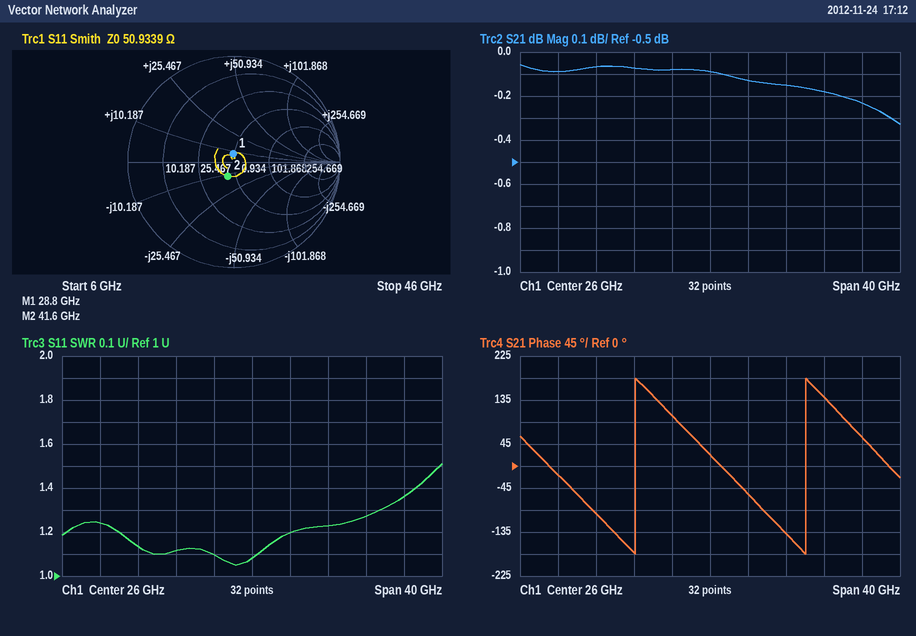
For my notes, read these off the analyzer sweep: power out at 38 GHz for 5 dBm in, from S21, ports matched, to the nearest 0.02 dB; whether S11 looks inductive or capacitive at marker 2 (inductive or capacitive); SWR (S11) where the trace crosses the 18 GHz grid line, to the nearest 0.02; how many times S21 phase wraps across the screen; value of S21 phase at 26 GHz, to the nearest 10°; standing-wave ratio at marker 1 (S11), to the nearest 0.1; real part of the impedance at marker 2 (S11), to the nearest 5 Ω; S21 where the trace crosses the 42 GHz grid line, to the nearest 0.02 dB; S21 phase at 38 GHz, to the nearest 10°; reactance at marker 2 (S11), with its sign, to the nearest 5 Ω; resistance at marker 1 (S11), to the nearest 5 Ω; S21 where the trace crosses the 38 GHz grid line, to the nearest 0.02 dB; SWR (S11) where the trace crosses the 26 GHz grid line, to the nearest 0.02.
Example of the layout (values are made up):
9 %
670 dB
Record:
4.82 dBm
capacitive
1.12
2
20°
1.2
45 Ω
-0.24 dB
140°
-10 Ω
50 Ω
-0.18 dB
1.08
